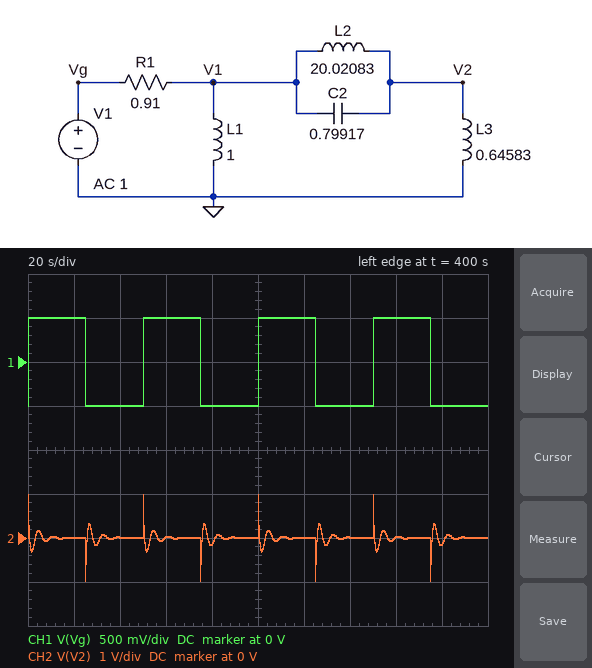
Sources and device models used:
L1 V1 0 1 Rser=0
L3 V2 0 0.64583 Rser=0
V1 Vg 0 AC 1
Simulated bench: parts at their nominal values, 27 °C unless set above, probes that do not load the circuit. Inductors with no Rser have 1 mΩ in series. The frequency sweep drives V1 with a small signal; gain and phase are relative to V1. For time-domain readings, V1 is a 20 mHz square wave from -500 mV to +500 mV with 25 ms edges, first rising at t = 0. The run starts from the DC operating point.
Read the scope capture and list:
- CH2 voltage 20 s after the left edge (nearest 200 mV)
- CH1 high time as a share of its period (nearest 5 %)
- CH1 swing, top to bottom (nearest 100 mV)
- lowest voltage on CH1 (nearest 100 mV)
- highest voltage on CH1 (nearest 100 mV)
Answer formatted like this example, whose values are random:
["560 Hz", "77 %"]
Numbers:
["0 V", "50 %", "1.0 V", "-500 mV", "500 mV"]
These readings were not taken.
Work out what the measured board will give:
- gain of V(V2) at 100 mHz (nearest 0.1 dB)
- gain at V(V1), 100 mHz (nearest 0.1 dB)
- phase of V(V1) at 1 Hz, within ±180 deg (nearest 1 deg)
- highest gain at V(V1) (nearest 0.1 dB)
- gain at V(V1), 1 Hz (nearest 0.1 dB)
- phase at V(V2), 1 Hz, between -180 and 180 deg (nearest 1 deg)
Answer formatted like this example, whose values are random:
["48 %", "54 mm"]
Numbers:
["-16.6 dB", "-2.9 dB", "21 deg", "0 dB", "-0.6 dB", "21 deg"]
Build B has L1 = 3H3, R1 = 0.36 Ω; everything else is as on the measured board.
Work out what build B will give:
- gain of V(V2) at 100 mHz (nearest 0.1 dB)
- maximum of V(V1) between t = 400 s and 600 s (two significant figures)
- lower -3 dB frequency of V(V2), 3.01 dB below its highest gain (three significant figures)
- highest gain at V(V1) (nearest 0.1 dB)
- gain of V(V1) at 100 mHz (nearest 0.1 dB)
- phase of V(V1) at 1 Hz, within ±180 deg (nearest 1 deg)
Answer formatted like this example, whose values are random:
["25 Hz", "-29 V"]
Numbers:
["-13.7 dB", "950 mV", "194 mHz", "0 dB", "0 dB", "6 deg"]
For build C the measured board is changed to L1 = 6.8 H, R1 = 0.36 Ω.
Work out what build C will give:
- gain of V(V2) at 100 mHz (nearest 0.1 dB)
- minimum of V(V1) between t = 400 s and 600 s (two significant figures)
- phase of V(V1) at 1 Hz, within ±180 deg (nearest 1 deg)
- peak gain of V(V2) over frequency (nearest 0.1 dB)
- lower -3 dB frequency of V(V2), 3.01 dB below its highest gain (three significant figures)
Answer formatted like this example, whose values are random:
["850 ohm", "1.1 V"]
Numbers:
["-13.7 dB", "-880 mV", "6 deg", "8.2 dB", "196 mHz"]
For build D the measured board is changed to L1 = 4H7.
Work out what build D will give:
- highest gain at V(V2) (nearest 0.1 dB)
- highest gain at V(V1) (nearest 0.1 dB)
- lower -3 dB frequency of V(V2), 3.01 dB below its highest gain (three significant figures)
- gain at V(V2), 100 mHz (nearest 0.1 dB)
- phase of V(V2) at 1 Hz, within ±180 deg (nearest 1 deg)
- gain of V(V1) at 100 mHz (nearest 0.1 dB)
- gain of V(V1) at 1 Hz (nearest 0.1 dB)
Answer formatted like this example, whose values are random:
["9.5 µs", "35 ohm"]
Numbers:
["0.8 dB", "0 dB", "180 mHz", "-13.8 dB", "15 deg", "-0.1 dB", "-0.3 dB"]
